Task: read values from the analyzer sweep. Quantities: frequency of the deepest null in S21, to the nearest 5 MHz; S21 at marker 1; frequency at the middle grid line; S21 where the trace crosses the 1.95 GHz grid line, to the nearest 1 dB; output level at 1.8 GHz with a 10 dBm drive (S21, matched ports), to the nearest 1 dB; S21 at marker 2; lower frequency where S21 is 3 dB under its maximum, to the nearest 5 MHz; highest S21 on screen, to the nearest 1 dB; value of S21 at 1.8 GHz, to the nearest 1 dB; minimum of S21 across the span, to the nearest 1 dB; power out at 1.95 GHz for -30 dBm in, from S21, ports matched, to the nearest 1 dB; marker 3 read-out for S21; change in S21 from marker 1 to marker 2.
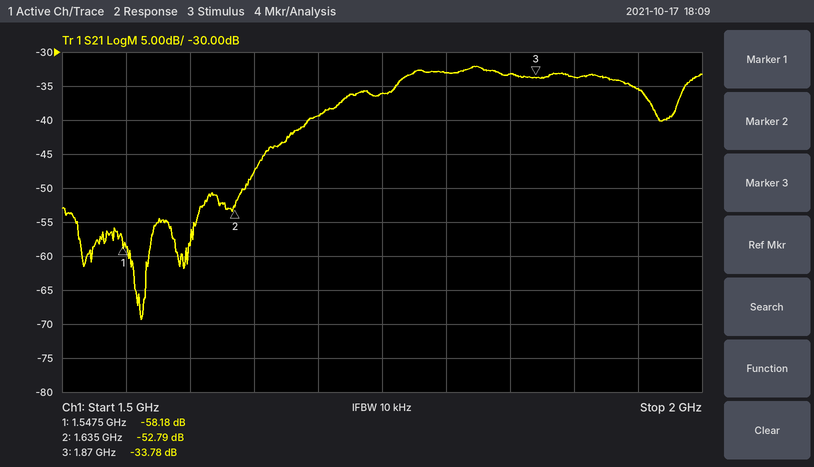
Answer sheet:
1.560 GHz
-58.18 dB
1.75 GHz
-35 dB
-23 dBm
-52.79 dB
1.760 GHz
-32 dB
-33 dB
-69 dB
-65 dBm
-33.78 dB
5.39 dB
